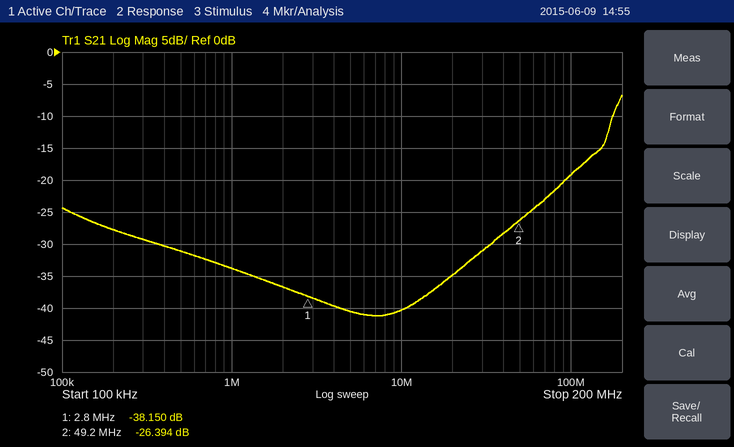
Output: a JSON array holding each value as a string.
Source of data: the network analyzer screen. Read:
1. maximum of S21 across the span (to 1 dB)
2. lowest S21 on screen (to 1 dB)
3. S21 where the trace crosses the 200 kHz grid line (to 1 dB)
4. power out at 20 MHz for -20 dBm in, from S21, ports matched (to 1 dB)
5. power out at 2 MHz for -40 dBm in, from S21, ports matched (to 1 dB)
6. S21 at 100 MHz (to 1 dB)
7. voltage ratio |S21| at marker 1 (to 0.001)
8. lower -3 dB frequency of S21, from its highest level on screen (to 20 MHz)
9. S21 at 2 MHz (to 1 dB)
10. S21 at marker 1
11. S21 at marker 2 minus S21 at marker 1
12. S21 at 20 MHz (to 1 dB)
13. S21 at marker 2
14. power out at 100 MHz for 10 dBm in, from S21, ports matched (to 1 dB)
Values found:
["-7 dB", "-41 dB", "-28 dB", "-55 dBm", "-77 dBm", "-19 dB", "0.012", "180 MHz", "-37 dB", "-38.150 dB", "11.756 dB", "-35 dB", "-26.394 dB", "-9 dBm"]
